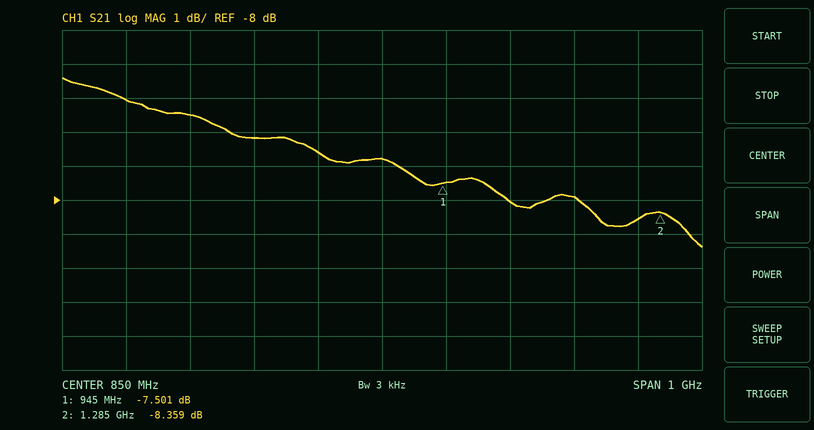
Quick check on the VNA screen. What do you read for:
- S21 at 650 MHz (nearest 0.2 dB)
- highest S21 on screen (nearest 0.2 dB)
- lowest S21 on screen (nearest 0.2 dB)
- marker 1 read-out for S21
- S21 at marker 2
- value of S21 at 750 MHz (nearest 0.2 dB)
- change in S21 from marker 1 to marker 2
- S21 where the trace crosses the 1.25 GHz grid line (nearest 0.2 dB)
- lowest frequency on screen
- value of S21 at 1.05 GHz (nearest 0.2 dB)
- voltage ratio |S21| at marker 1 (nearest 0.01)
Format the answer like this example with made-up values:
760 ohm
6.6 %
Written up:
-6.2 dB
-4.4 dB
-9.4 dB
-7.501 dB
-8.359 dB
-6.6 dB
-0.858 dB
-8.6 dB
350 MHz
-8.0 dB
0.42
